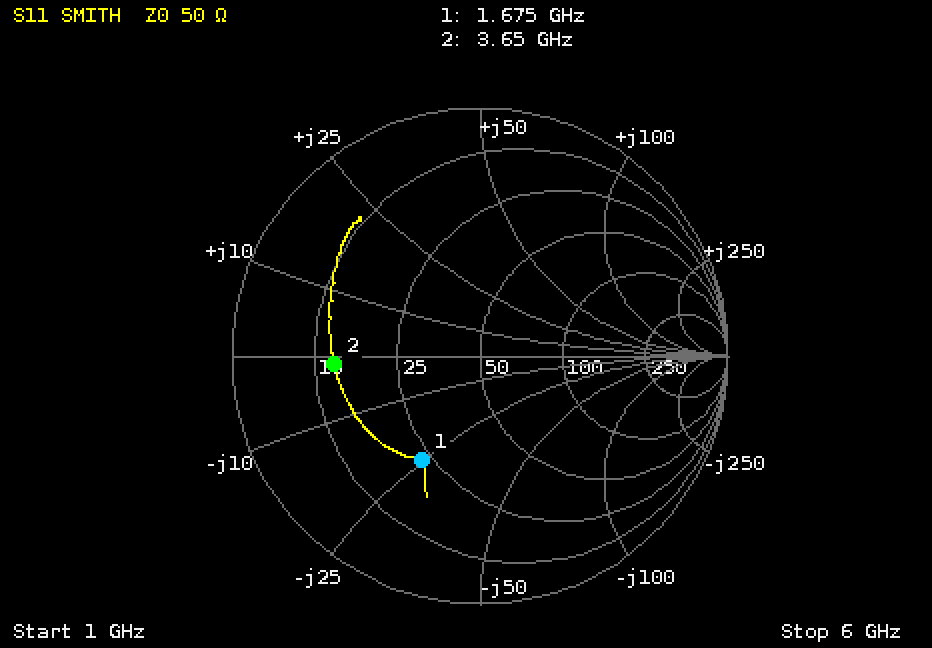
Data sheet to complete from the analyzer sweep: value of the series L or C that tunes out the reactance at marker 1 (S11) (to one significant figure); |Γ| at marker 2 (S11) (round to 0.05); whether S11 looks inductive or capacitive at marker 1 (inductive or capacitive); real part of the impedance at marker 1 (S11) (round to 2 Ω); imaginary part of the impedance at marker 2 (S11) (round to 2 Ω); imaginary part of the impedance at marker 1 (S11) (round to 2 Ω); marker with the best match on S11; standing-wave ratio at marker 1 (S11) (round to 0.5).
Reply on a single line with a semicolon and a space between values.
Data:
2 nH; 0.60; capacitive; 22 Ω; -2 Ω; -24 Ω; marker 1; 3.0
